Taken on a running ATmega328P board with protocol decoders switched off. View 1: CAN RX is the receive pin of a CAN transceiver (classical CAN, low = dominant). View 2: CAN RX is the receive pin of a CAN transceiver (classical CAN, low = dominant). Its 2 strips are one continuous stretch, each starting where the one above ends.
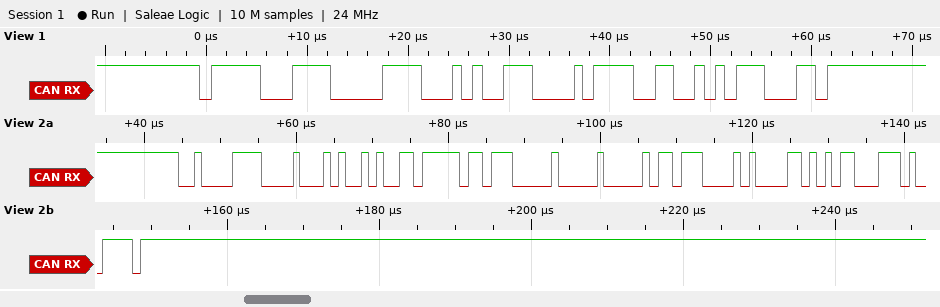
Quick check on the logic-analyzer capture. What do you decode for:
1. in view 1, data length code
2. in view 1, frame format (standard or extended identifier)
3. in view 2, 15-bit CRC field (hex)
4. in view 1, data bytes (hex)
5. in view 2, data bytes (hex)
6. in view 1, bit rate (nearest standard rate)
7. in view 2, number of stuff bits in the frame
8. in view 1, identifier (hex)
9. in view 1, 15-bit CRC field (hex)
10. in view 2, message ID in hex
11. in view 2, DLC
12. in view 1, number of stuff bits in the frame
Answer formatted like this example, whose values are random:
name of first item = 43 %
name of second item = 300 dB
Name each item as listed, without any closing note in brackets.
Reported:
in view 1, data length code = 3
in view 1, frame format = standard
in view 2, 15-bit CRC field = 0x63A7
in view 1, data bytes = 8A 70 BC
in view 2, data bytes = A5 37 F7 00 00 DC 28 6A
in view 1, bit rate = 1000 kbit/s
in view 2, number of stuff bits in the frame = 4
in view 1, identifier = 0x7CF
in view 1, 15-bit CRC field = 0x6571
in view 2, message ID in hex = 0x21E
in view 2, DLC = 8
in view 1, number of stuff bits in the frame = 2
